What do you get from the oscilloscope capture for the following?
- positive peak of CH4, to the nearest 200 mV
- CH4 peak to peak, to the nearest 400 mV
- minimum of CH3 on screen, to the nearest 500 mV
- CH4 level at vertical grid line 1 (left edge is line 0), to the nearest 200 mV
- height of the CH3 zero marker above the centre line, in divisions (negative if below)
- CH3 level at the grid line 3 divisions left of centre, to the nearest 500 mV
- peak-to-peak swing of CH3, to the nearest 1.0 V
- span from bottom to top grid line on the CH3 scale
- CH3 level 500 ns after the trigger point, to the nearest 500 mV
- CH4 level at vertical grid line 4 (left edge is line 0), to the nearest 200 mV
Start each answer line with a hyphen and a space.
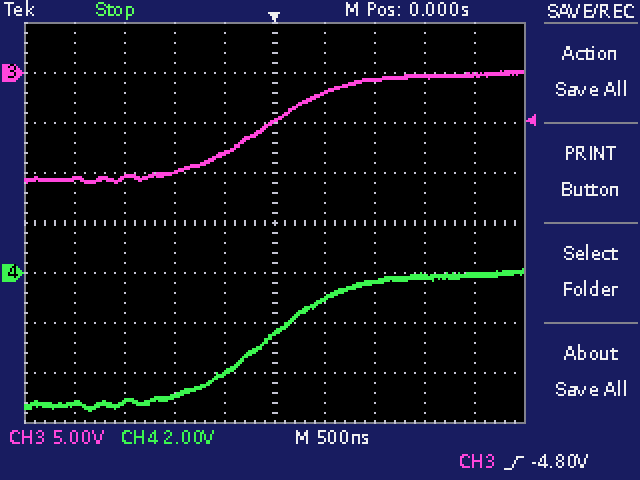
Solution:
- 200 mV
- 5.6 V
- -11.0 V
- -5.2 V
- +3.0 div
- -10.5 V
- 11.0 V
- 40 V
- -2.0 V
- -4.0 V
